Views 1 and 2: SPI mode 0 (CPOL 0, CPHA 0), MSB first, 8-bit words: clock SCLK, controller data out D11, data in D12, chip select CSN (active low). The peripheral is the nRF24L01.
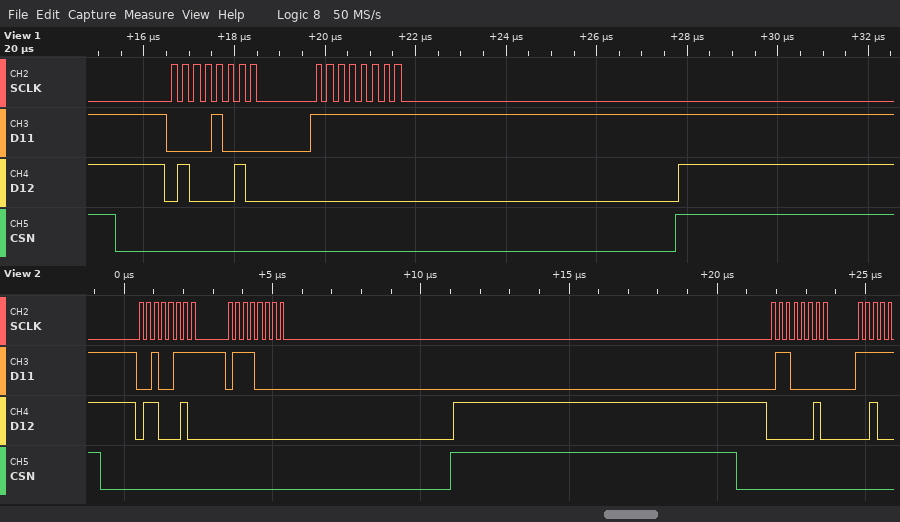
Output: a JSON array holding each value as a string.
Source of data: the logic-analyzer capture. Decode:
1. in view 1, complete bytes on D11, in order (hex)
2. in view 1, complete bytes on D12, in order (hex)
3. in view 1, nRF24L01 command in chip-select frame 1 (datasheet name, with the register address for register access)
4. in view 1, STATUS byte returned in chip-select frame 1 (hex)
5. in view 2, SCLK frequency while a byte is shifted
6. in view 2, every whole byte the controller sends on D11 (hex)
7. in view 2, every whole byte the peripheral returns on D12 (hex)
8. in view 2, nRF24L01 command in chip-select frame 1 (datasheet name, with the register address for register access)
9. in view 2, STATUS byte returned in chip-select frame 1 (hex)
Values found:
["08 FF", "42 00", "R_REGISTER 0x08", "0x42", "4 MHz", "27 70 60", "62 00 02", "W_REGISTER 0x07", "0x62"]
